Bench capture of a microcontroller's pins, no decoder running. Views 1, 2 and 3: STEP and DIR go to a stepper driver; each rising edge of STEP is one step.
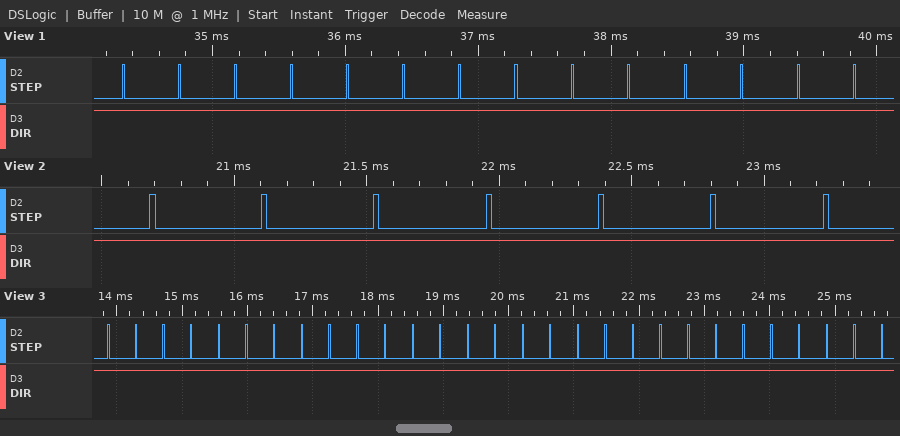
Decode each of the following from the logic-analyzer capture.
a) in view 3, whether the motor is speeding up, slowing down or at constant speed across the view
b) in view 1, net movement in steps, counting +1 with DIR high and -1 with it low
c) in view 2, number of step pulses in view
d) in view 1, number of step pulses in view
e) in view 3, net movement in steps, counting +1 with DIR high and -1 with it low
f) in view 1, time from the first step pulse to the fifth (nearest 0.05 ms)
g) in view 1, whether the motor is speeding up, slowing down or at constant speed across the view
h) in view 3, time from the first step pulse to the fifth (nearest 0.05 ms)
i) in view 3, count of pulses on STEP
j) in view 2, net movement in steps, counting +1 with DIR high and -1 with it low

constant speed
+14
7
14
+29
1.70 ms
constant speed
1.70 ms
29
+7
